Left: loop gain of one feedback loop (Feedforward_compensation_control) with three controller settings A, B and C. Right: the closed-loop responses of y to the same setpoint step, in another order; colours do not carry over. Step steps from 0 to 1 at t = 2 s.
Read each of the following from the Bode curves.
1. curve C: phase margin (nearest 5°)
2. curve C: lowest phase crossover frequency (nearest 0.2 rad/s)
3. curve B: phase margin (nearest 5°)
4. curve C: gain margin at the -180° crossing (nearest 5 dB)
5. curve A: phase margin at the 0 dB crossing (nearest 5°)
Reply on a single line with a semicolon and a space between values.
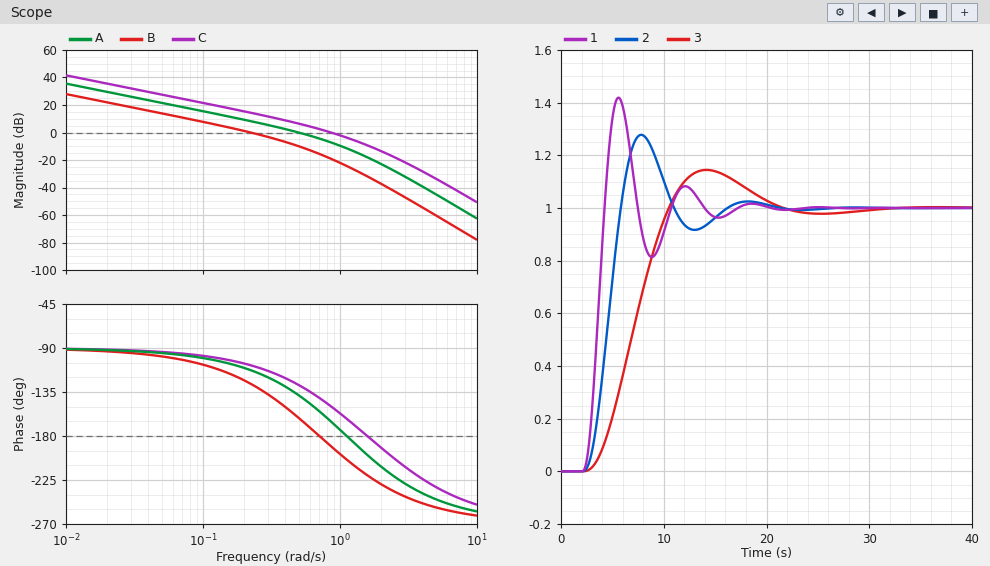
30°; 1.6 rad/s; 55°; 10 dB; 40°
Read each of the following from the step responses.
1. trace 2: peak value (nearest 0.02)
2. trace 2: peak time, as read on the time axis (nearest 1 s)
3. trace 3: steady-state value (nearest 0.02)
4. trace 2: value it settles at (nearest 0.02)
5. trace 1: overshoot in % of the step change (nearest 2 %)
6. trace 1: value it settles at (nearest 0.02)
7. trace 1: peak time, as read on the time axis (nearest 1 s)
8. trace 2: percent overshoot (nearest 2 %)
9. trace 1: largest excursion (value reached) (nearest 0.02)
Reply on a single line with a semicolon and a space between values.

1.28; 8 s; 1.00; 1.00; 42 %; 1.00; 6 s; 28 %; 1.42
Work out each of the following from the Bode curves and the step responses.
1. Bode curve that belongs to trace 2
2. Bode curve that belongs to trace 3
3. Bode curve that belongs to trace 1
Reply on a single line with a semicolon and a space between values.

A; B; C
